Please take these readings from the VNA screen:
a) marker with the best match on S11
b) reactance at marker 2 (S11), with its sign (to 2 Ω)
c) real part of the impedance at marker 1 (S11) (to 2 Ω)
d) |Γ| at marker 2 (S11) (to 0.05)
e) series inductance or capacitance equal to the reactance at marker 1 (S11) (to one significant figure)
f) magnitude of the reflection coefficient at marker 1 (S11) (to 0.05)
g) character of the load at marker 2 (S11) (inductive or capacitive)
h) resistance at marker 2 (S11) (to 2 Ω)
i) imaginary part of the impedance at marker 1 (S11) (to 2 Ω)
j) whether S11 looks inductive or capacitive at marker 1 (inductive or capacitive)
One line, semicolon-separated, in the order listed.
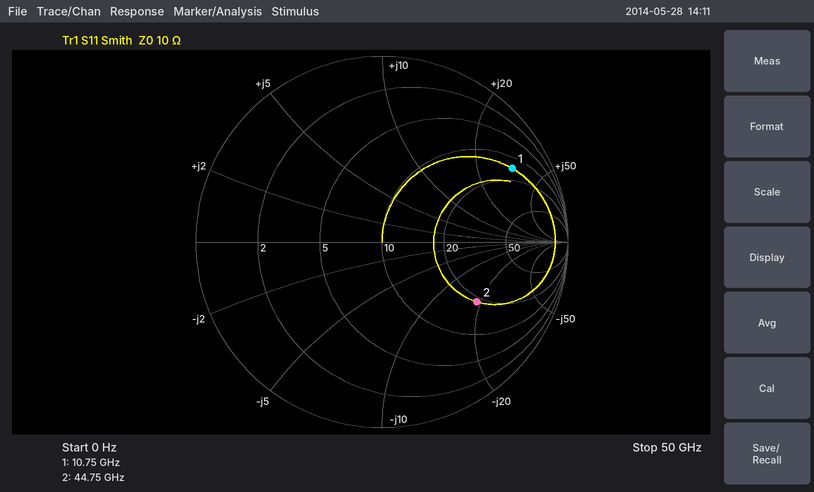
marker 2; -18 Ω; 14 Ω; 0.60; 500 pH; 0.80; capacitive; 18 Ω; +32 Ω; inductive
